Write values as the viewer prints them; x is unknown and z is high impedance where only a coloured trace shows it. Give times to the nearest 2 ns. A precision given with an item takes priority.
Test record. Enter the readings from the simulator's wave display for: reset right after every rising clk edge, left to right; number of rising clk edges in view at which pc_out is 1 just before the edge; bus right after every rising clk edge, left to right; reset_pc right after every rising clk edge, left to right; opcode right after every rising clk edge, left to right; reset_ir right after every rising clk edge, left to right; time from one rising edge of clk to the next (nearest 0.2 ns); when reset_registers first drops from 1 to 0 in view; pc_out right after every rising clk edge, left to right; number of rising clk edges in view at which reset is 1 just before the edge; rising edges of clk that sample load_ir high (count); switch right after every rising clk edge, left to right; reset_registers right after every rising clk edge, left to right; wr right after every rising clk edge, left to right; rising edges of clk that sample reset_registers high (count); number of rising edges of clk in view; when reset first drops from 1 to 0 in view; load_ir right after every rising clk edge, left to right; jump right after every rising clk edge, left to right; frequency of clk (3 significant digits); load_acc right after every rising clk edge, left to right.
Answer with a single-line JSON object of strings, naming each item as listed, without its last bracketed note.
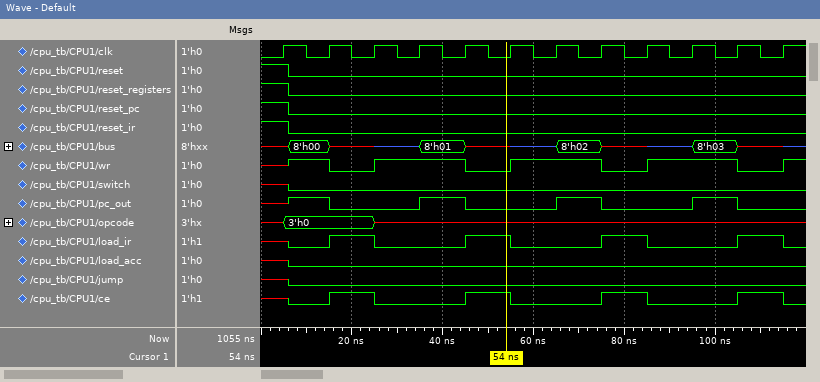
{"reset right after every rising clk edge, left to right": "1 0 0 0 0 0 0 0 0 0 0 0", "number of rising clk edges in view at which pc_out is 1 just before the edge": "4", "bus right after every rising clk edge, left to right": "x, x, z, 8'h01, x, z, 8'h02, x, z, 8'h03, x, z", "reset_pc right after every rising clk edge, left to right": "1 0 0 0 0 0 0 0 0 0 0 0", "opcode right after every rising clk edge, left to right": "3'h0, 3'h0, x, x, x, x, x, x, x, x, x, x", "reset_ir right after every rising clk edge, left to right": "1 0 0 0 0 0 0 0 0 0 0 0", "time from one rising edge of clk to the next": "10 ns", "when reset_registers first drops from 1 to 0 in view": "6 ns", "pc_out right after every rising clk edge, left to right": "x 0 0 1 0 0 1 0 0 1 0 0", "number of rising clk edges in view at which reset is 1 just before the edge": "1", "rising edges of clk that sample load_ir high": "4", "switch right after every rising clk edge, left to right": "x 0 0 0 0 0 0 0 0 0 0 0", "reset_registers right after every rising clk edge, left to right": "1 0 0 0 0 0 0 0 0 0 0 0", "wr right after every rising clk edge, left to right": "x 0 1 1 0 1 1 0 1 1 0 1", "rising edges of clk that sample reset_registers high": "1", "number of rising edges of clk in view": "12", "when reset first drops from 1 to 0 in view": "6 ns", "load_ir right after every rising clk edge, left to right": "x 1 0 0 1 0 0 1 0 0 1 0", "jump right after every rising clk edge, left to right": "x 0 0 0 0 0 0 0 0 0 0 0", "frequency of clk": "100 MHz", "load_acc right after every rising clk edge, left to right": "x 0 0 0 0 0 0 0 0 0 0 0"}
